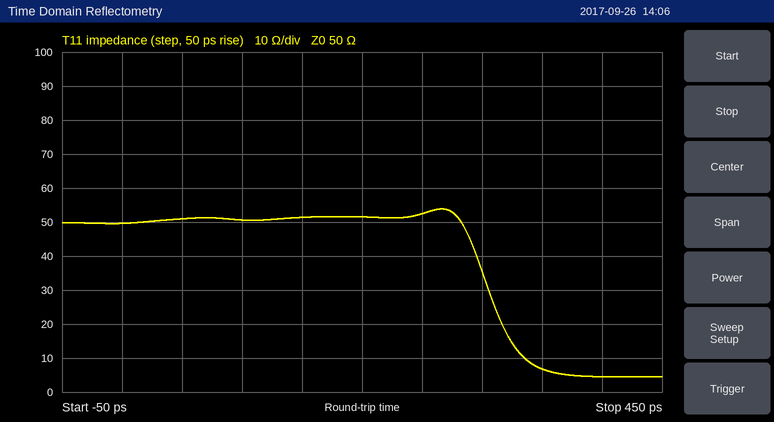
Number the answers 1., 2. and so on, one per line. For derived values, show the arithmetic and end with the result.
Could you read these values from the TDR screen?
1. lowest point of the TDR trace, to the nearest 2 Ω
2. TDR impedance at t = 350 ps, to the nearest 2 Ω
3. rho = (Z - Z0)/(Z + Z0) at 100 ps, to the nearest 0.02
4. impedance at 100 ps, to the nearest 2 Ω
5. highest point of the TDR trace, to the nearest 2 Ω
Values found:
1. 4 Ω
2. 6 Ω
3. (50 − 50)/(50 + 50) ≈ 0.00
4. 50 Ω
5. 54 Ω
